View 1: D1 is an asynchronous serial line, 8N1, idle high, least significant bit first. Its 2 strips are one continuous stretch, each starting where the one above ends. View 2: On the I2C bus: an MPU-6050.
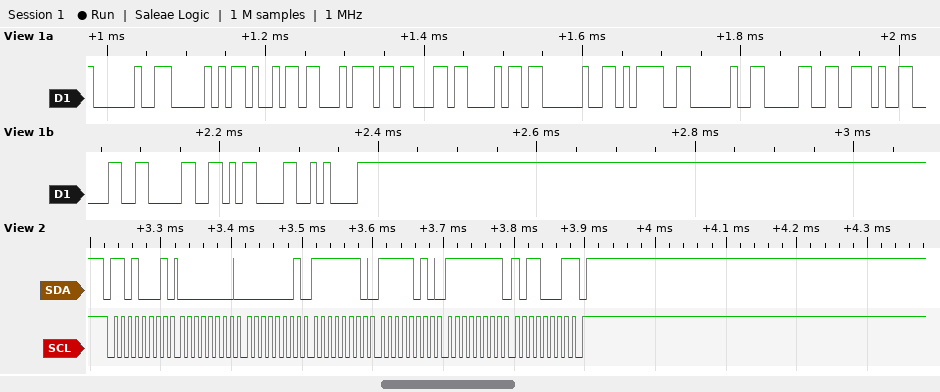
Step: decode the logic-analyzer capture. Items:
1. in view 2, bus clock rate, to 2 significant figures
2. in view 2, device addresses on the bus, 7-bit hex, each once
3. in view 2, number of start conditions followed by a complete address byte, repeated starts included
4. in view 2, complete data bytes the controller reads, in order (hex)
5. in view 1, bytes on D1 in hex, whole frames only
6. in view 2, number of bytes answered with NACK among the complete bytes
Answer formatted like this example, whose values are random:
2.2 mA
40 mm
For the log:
100 kHz
0x68
1
00 01 FE FA FF B1
20 50 69 74 63 68 20 3D 20 30 2E 30 30 0D 0A
1
